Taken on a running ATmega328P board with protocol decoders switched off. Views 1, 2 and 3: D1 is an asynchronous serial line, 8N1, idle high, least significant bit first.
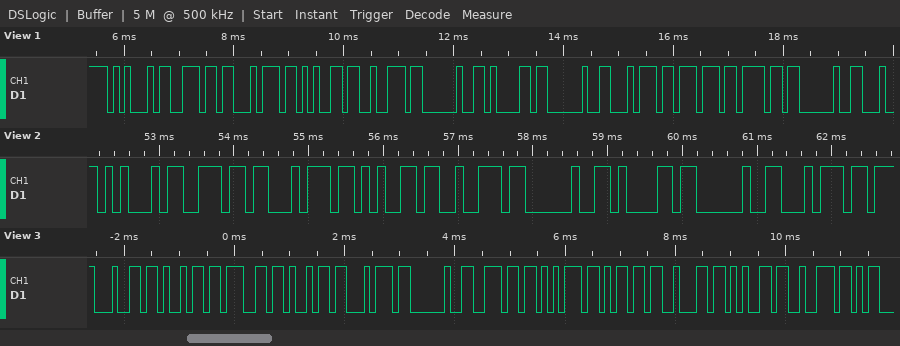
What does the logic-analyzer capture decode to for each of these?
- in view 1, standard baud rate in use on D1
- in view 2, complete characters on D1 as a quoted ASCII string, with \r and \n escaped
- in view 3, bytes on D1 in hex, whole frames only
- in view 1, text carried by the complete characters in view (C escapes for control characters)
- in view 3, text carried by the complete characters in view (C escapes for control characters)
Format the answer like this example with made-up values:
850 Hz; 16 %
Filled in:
9600 baud; "Enter a t"; 64 69 67 69 74 20 6E 75 6D 62 65 72; "Enter a two "; "digit number"
